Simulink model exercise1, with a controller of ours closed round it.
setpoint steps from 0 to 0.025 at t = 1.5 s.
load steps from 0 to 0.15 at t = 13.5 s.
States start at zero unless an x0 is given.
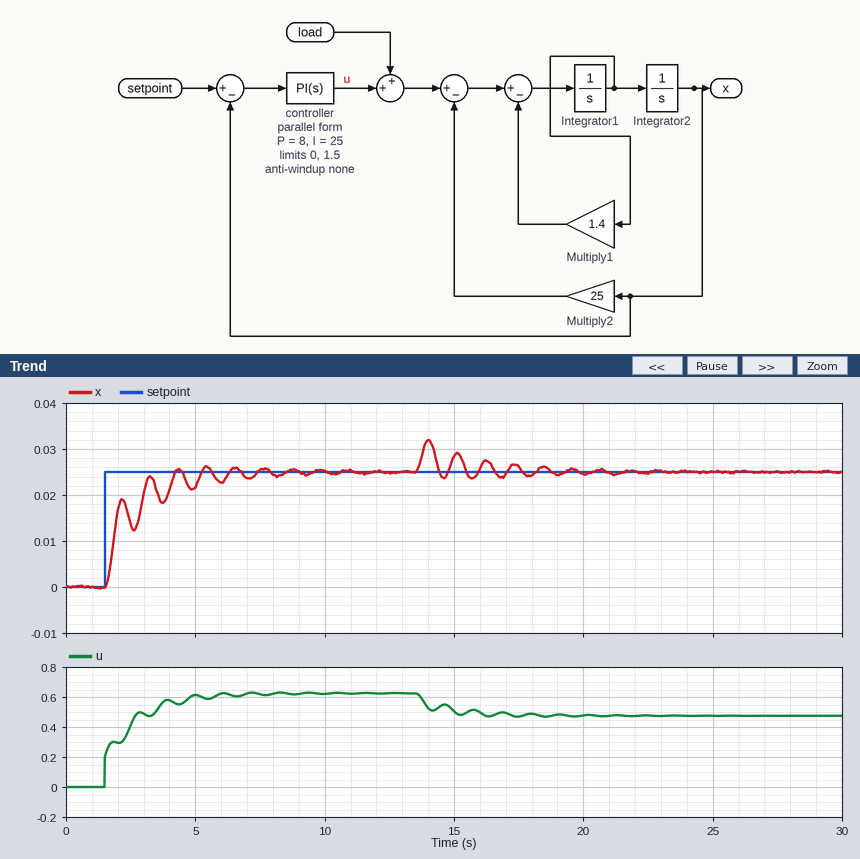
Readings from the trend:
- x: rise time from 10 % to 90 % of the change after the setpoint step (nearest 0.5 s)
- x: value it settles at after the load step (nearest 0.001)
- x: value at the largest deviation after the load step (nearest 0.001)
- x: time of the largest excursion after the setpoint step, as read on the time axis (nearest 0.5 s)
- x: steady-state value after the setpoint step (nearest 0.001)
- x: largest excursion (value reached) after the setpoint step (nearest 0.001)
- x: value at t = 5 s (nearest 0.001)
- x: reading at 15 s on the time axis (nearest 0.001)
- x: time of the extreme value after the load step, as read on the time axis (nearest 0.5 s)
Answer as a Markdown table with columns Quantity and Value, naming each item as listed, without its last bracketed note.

| Quantity | Value |
|---|---|
| x: rise time from 10 % to 90 % of the change after the setpoint step | 1.5 s |
| x: value it settles at after the load step | 0.025 |
| x: value at the largest deviation after the load step | 0.032 |
| x: time of the largest excursion after the setpoint step, as read on the time axis | 5.5 s |
| x: steady-state value after the setpoint step | 0.025 |
| x: largest excursion (value reached) after the setpoint step | 0.026 |
| x: value at t = 5 s | 0.022 |
| x: reading at 15 s on the time axis | 0.028 |
| x: time of the extreme value after the load step, as read on the time axis | 14.0 s |
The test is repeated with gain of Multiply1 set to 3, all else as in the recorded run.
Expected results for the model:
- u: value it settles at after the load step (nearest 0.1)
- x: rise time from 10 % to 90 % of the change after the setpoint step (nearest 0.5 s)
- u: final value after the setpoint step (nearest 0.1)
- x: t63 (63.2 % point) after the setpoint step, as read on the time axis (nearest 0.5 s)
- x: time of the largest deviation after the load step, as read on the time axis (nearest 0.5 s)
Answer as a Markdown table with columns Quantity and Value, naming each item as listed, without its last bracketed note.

| Quantity | Value |
|---|---|
| u: value it settles at after the load step | 0.5 |
| x: rise time from 10 % to 90 % of the change after the setpoint step | 2.5 s |
| u: final value after the setpoint step | 0.6 |
| x: t63 (63.2 % point) after the setpoint step, as read on the time axis | 2.0 s |
| x: time of the largest deviation after the load step, as read on the time axis | 14.0 s |
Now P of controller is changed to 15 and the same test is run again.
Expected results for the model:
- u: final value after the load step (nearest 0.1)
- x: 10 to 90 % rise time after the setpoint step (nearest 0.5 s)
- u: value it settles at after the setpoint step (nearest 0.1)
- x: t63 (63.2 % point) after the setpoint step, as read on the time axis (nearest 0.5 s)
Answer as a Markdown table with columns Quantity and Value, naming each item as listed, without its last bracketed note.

| Quantity | Value |
|---|---|
| u: final value after the load step | 0.5 |
| x: 10 to 90 % rise time after the setpoint step | 1.5 s |
| u: value it settles at after the setpoint step | 0.6 |
| x: t63 (63.2 % point) after the setpoint step, as read on the time axis | 2.0 s |
